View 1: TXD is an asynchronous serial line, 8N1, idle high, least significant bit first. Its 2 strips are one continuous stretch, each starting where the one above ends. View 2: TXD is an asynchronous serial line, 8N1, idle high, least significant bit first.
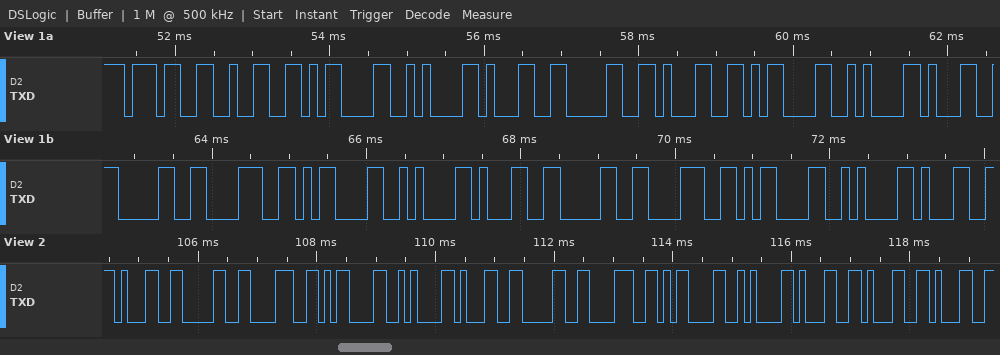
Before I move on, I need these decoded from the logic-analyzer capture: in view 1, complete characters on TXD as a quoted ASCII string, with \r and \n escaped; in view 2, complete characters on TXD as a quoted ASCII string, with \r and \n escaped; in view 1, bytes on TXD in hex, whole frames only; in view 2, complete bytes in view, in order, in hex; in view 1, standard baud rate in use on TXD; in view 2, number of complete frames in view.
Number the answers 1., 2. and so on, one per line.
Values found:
1. "72\r\n101\r\n108\r\n108\r\n1"
2. "108\r\n108\r\n111"
3. 37 32 0D 0A 31 30 31 0D 0A 31 30 38 0D 0A 31 30 38 0D 0A 31
4. 0x31 0x30 0x38 0x0D 0x0A 0x31 0x30 0x38 0x0D 0x0A 0x31 0x31 0x31
5. 9600 baud
6. 13
